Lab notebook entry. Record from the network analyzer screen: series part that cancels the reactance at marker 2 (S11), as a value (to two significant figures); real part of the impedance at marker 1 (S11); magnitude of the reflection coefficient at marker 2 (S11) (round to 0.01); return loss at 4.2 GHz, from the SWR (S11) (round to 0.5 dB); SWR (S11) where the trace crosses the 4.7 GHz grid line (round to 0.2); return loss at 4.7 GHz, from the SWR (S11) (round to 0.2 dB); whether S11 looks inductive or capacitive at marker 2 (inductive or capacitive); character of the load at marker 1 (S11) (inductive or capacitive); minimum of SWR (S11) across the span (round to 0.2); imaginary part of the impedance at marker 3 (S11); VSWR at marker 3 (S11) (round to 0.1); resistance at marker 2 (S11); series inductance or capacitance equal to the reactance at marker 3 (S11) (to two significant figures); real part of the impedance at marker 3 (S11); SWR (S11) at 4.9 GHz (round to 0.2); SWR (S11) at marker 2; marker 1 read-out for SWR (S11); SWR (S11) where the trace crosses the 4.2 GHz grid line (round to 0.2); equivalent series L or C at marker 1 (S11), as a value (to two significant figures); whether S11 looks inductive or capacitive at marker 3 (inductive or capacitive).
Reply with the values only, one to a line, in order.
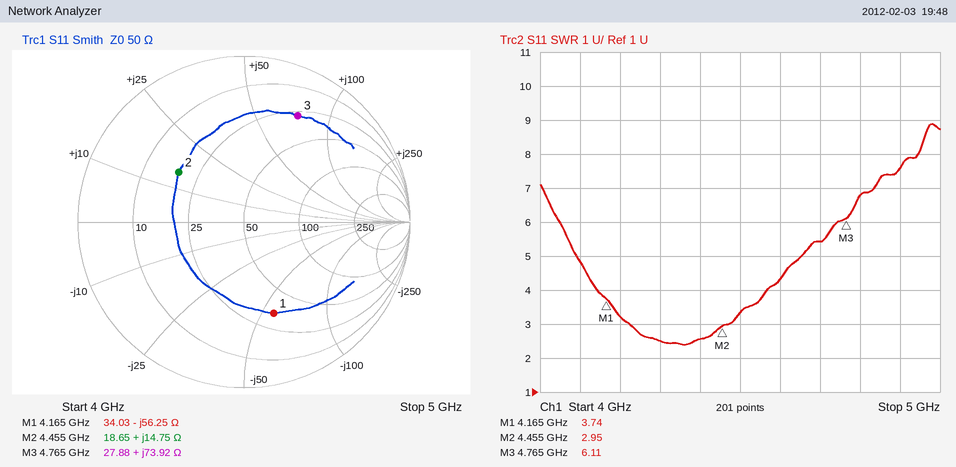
2.4 pF
34.03 Ω
0.49
5.5 dB
5.4
3.2 dB
inductive
capacitive
2.4
+73.92 Ω
6.1
18.65 Ω
2.5 nH
27.88 Ω
7.6
2.95
3.74
3.2
680 fF
inductive
